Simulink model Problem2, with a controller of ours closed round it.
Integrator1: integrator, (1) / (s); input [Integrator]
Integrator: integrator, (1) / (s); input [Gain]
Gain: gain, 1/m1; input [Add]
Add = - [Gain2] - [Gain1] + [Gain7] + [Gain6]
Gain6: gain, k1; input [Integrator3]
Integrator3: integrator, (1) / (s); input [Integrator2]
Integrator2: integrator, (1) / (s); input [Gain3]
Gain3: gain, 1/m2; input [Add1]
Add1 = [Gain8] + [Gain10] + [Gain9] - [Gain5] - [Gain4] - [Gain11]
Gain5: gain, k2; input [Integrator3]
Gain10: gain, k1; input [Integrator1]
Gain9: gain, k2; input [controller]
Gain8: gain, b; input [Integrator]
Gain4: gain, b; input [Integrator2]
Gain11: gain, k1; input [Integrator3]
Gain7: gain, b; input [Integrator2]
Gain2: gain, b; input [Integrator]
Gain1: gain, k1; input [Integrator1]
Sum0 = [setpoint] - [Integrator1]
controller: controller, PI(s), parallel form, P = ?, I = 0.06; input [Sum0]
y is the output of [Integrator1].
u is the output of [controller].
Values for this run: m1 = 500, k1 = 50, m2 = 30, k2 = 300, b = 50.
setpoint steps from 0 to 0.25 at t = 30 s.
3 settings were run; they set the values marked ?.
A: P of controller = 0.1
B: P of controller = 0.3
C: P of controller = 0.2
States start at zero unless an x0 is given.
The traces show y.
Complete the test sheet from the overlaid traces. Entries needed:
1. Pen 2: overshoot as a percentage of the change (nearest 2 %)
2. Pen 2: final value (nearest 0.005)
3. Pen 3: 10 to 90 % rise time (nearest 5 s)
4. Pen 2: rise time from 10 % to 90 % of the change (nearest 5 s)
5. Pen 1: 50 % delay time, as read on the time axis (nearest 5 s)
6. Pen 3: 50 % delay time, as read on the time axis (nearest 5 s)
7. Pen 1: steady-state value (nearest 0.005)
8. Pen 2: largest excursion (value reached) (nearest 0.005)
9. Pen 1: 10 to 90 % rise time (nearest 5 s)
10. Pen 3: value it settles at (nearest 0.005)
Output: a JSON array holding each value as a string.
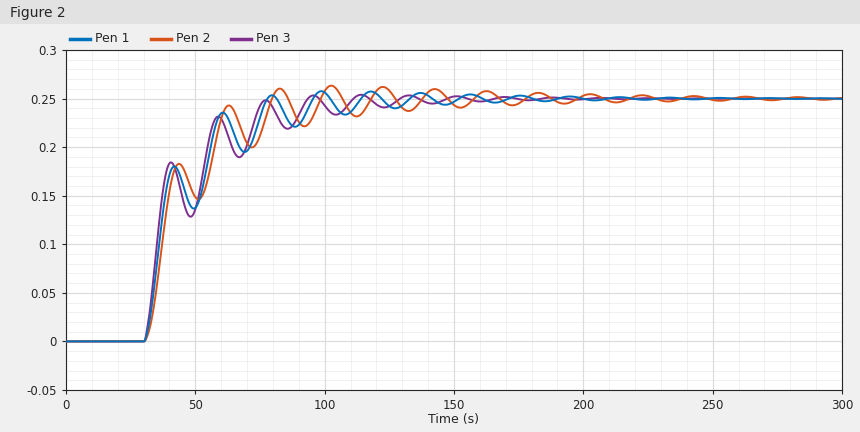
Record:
["6 %", "0.250", "25 s", "25 s", "35 s", "35 s", "0.250", "0.265", "25 s", "0.250"]
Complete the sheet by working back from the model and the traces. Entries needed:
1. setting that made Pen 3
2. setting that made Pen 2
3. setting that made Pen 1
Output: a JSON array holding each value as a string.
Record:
["B", "A", "C"]
